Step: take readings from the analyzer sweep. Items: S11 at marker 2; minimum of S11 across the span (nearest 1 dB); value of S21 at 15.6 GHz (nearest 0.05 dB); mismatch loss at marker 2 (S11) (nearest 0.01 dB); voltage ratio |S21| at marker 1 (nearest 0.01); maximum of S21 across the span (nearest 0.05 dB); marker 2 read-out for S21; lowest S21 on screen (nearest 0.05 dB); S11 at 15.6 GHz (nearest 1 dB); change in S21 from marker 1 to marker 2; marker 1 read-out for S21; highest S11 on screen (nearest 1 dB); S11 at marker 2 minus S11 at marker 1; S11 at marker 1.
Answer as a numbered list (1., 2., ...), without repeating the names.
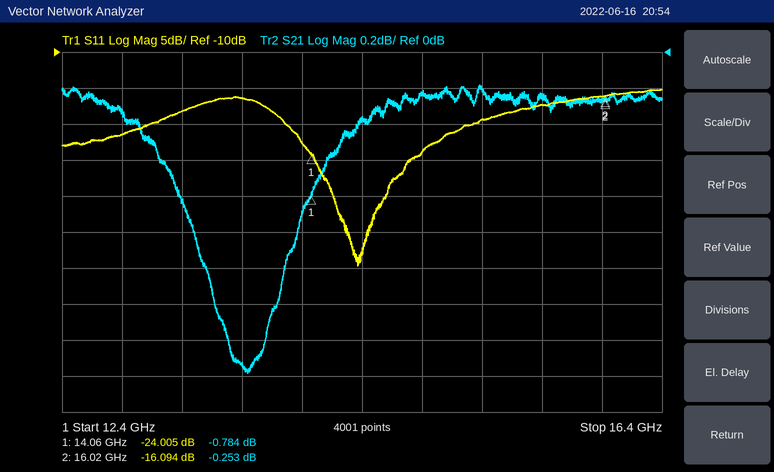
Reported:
1. -16.094 dB
2. -40 dB
3. -0.25 dB
4. 0.11 dB
5. 0.91
6. -0.20 dB
7. -0.253 dB
8. -1.80 dB
9. -17 dB
10. 0.531 dB
11. -0.784 dB
12. -15 dB
13. 7.911 dB
14. -24.005 dB
